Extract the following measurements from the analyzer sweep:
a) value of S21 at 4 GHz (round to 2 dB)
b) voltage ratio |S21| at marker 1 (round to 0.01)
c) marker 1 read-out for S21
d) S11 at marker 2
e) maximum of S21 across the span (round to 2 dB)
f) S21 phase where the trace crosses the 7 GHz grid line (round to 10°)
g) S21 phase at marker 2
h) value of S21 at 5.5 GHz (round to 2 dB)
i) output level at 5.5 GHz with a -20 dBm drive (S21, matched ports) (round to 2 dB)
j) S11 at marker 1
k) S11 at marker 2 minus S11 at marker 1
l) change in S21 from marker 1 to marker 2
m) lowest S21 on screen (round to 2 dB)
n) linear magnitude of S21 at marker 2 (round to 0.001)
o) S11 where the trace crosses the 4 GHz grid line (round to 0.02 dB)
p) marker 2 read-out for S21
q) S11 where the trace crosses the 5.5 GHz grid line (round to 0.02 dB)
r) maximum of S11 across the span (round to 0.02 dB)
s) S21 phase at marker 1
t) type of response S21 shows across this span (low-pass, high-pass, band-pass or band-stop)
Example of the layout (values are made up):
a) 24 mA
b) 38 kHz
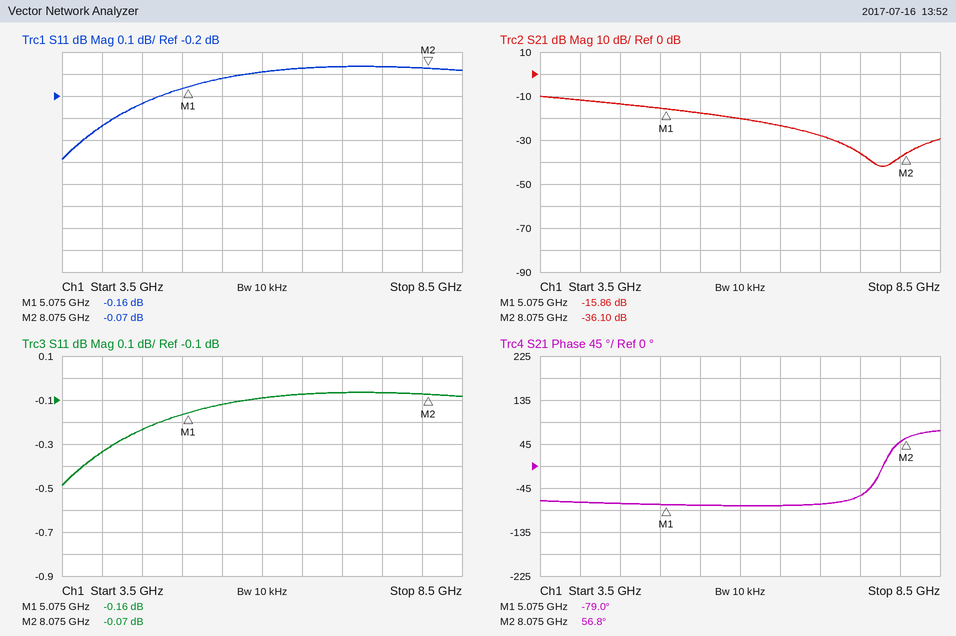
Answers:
a) -12 dB
b) 0.16
c) -15.86 dB
d) -0.07 dB
e) -10 dB
f) -80°
g) 56.8°
h) -18 dB
i) -38 dBm
j) -0.16 dB
k) 0.09 dB
l) -20.24 dB
m) -42 dB
n) 0.016
o) -0.34 dB
p) -36.10 dB
q) -0.12 dB
r) -0.06 dB
s) -79.0°
t) low-pass
